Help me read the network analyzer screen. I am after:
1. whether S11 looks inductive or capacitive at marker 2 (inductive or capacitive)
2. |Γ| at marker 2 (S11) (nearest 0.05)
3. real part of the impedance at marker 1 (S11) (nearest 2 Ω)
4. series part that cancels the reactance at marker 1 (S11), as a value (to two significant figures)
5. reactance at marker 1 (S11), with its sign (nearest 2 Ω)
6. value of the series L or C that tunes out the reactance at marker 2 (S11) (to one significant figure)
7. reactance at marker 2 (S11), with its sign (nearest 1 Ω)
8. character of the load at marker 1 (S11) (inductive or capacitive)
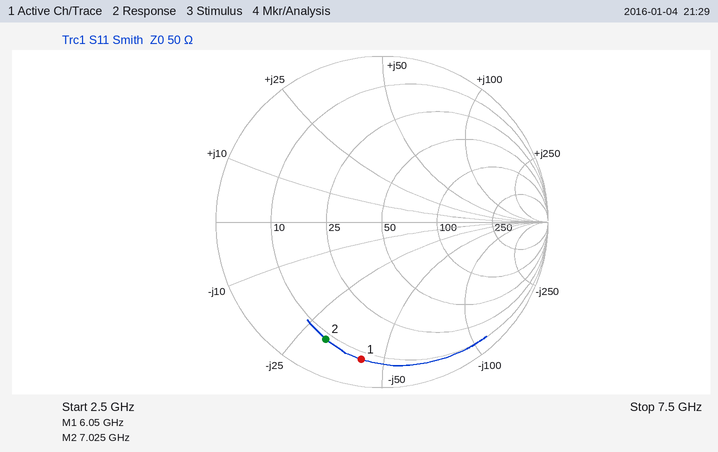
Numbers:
capacitive
0.80
8 Ω
1.1 nH
-42 Ω
700 pH
-31 Ω
capacitive
